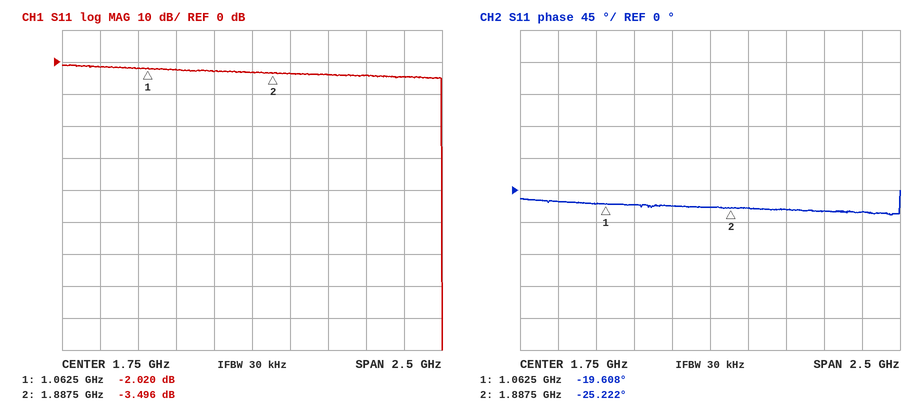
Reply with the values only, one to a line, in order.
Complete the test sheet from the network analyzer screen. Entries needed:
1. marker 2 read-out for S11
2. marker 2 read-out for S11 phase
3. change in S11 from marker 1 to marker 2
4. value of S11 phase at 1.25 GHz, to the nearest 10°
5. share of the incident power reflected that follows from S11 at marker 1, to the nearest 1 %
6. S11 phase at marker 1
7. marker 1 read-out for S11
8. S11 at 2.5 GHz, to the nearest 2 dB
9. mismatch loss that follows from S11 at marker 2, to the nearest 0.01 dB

-3.496 dB
-25.222°
-1.476 dB
-20°
63 %
-19.608°
-2.020 dB
-4 dB
2.57 dB
